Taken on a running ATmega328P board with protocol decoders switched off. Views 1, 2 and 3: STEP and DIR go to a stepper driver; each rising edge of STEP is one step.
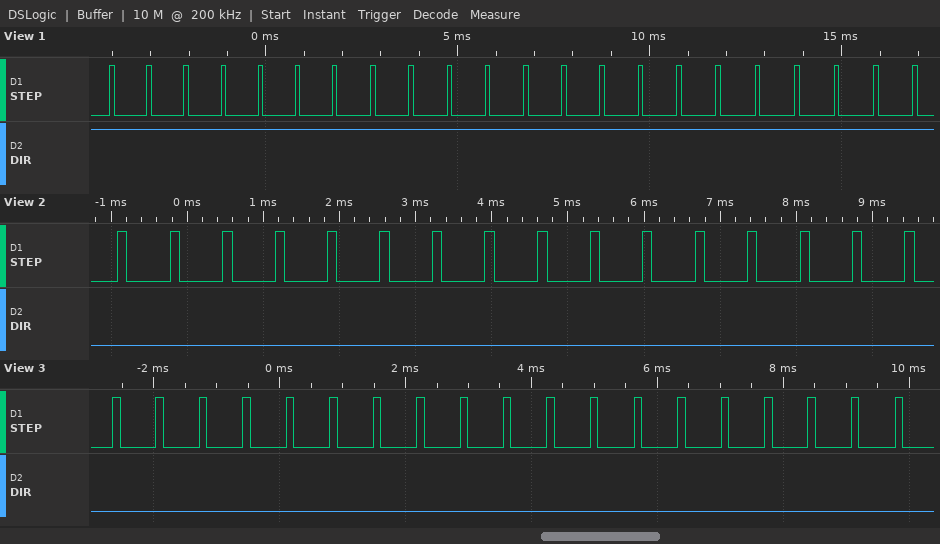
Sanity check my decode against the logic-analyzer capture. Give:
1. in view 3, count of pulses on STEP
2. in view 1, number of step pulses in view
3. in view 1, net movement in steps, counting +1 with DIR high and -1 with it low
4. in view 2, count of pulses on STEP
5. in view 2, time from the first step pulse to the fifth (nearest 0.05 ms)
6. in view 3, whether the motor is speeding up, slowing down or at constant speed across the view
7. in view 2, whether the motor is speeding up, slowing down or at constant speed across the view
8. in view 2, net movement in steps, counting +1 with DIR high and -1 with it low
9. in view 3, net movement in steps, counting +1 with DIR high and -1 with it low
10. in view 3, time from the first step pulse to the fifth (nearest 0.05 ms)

19
22
+22
16
2.75 ms
constant speed
constant speed
-16
-19
2.75 ms
